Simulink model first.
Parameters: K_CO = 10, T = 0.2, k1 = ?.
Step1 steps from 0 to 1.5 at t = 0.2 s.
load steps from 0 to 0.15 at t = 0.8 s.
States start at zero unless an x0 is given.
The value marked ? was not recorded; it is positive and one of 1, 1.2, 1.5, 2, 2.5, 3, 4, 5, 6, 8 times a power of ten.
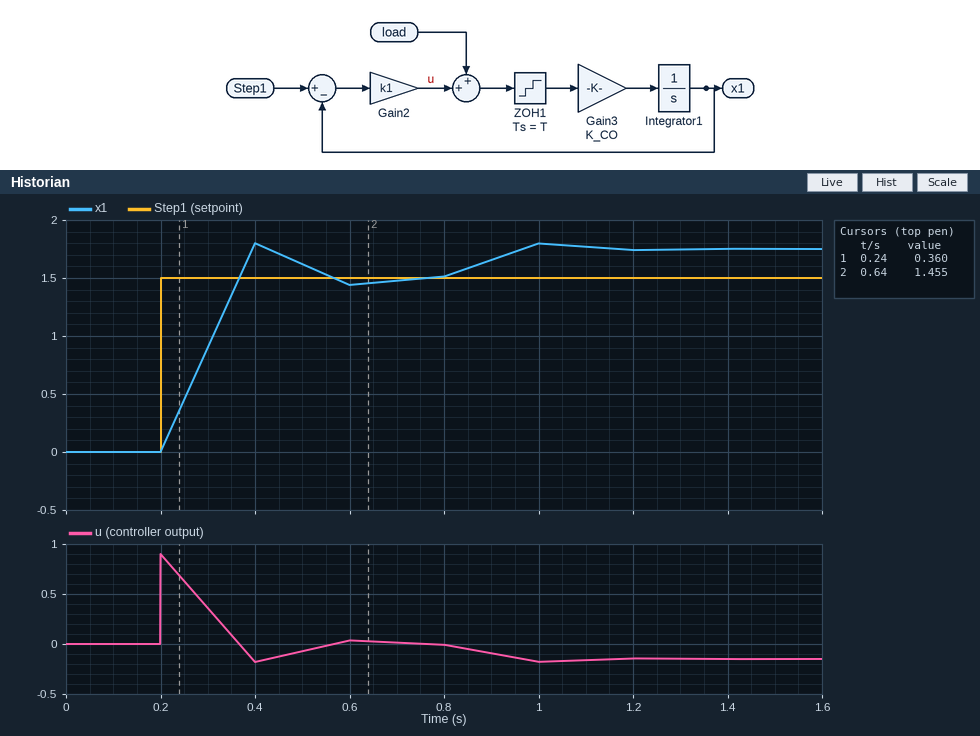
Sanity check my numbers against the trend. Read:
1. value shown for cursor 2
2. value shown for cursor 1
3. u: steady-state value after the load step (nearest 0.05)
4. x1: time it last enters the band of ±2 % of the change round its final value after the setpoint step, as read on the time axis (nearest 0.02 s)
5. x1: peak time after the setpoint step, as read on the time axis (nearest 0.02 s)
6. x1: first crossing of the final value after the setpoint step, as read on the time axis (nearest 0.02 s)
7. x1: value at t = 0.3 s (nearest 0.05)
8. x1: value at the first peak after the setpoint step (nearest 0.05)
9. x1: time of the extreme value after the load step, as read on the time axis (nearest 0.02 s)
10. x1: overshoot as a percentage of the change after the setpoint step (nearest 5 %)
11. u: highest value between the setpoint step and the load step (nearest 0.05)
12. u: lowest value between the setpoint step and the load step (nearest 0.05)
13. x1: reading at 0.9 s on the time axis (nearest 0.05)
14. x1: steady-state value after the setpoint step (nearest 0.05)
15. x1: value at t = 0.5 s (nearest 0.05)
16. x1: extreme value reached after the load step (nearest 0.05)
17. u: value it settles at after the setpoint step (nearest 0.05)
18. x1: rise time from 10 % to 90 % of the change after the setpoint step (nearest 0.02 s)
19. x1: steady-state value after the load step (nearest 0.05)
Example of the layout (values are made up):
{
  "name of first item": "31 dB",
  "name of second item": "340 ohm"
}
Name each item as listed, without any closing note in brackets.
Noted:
{
  "value shown for cursor 2": "1.455",
  "value shown for cursor 1": "0.360",
  "u: steady-state value after the load step": "-0.15",
  "x1: time it last enters the band of ±2 % of the change round its final value after the setpoint step, as read on the time axis": "0.68 s",
  "x1: peak time after the setpoint step, as read on the time axis": "0.40 s",
  "x1: first crossing of the final value after the setpoint step, as read on the time axis": "0.36 s",
  "x1: value at t = 0.3 s": "0.90",
  "x1: value at the first peak after the setpoint step": "1.80",
  "x1: time of the extreme value after the load step, as read on the time axis": "1.00 s",
  "x1: overshoot as a percentage of the change after the setpoint step": "20 %",
  "u: highest value between the setpoint step and the load step": "0.90",
  "u: lowest value between the setpoint step and the load step": "-0.20",
  "x1: reading at 0.9 s on the time axis": "1.65",
  "x1: steady-state value after the setpoint step": "1.50",
  "x1: value at t = 0.5 s": "1.60",
  "x1: extreme value reached after the load step": "1.80",
  "u: value it settles at after the setpoint step": "0.00",
  "x1: rise time from 10 % to 90 % of the change after the setpoint step": "0.14 s",
  "x1: steady-state value after the load step": "1.75"
}
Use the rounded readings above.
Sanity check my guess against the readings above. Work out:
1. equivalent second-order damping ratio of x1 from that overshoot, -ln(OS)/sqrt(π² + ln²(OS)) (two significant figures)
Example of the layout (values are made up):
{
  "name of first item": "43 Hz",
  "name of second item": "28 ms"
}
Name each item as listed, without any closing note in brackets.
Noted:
{
  "equivalent second-order damping ratio of x1 from that overshoot, -ln(OS)/sqrt(π² + ln²(OS))": "0.46"
}
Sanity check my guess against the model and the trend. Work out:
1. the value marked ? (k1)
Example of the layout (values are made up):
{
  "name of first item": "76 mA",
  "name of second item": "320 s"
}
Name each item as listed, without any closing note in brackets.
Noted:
{
  "the value marked ?": "0.6"
}
